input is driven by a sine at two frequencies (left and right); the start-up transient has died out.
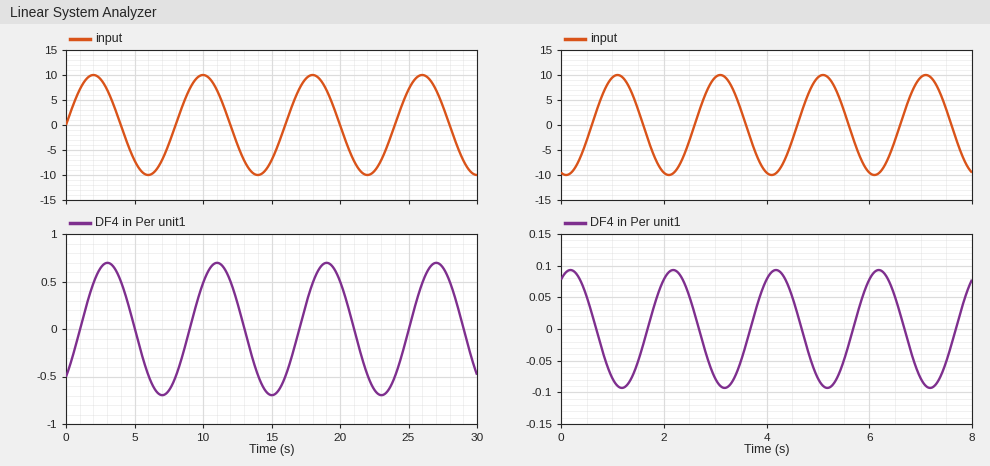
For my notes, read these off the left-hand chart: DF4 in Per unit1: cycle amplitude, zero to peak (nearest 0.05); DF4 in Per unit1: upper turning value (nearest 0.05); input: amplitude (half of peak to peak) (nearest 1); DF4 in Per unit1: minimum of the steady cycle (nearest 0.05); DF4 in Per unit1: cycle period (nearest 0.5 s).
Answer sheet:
0.70
0.70
10
-0.70
8.0 s
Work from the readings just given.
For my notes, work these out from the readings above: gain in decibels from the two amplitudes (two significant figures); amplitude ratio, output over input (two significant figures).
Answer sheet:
-23 dB
0.070
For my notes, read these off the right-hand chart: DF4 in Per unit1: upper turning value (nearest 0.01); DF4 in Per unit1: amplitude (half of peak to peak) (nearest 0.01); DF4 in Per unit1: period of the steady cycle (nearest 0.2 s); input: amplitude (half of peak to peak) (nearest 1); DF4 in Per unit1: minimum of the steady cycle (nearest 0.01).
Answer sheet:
0.09
0.09
2.0 s
10
-0.09
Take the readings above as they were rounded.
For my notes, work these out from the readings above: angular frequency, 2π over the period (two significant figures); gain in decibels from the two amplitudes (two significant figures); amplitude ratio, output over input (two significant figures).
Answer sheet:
3.1 rad/s
-41 dB
0.0090
